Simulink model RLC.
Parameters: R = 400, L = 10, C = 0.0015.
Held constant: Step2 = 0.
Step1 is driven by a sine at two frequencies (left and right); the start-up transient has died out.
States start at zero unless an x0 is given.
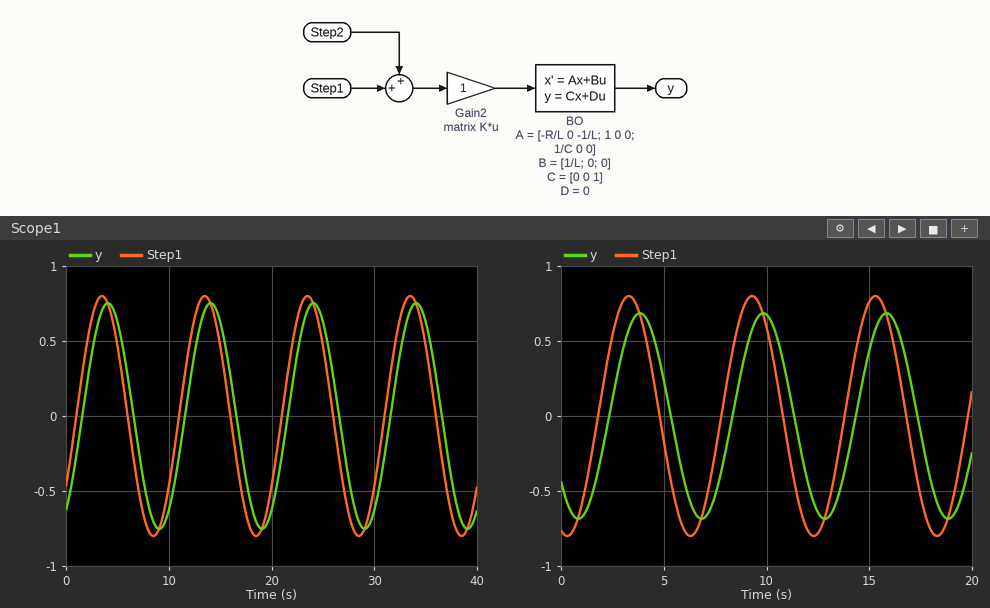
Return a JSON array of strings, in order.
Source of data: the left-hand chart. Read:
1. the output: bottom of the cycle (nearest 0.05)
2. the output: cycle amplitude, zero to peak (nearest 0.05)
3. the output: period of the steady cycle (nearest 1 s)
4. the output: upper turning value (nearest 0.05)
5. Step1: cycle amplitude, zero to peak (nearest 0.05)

["-0.75", "0.75", "10 s", "0.75", "0.80"]
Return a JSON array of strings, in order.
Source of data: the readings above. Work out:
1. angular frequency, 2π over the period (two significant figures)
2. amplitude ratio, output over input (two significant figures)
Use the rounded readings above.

["0.63 rad/s", "0.94"]
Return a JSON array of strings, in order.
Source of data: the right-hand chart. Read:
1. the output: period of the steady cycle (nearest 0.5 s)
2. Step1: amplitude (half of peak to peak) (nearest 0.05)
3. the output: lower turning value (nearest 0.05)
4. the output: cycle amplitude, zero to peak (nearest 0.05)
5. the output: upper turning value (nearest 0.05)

["6.0 s", "0.80", "-0.70", "0.70", "0.70"]
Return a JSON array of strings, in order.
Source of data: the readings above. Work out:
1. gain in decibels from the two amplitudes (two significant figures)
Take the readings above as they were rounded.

["-1.2 dB"]
